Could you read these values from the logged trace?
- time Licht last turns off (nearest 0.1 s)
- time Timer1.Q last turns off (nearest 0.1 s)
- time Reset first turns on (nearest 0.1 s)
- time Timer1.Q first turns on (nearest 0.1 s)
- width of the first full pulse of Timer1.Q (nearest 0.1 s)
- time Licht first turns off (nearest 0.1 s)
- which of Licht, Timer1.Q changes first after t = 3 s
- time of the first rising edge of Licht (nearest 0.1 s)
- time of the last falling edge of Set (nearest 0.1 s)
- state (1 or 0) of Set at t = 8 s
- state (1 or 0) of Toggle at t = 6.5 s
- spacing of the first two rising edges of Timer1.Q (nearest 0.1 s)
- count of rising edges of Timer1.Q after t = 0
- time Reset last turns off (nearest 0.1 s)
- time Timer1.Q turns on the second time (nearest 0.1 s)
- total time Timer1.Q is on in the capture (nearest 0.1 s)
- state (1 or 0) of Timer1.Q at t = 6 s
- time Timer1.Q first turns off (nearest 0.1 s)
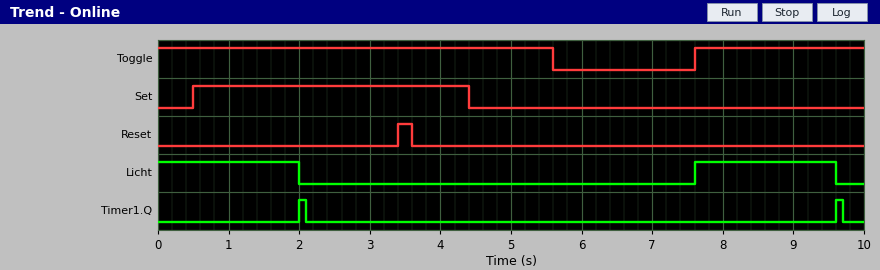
9.6 s
9.7 s
3.4 s
2.0 s
0.1 s
2.0 s
Licht
7.6 s
4.4 s
0
0
7.6 s
2
3.6 s
9.6 s
0.2 s
0
2.1 s
